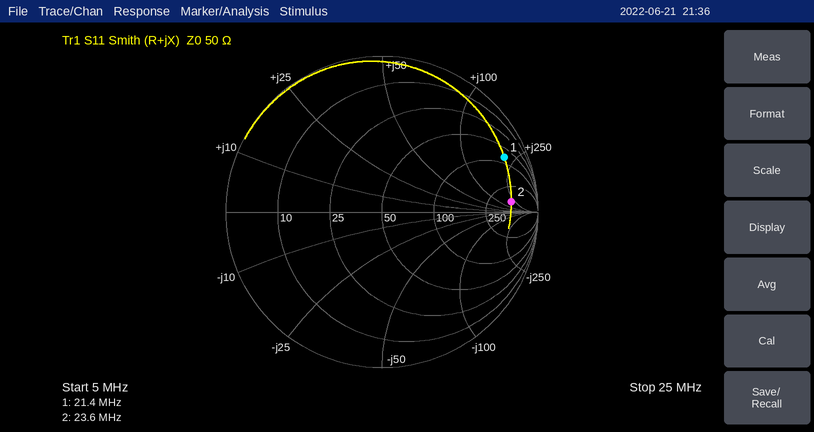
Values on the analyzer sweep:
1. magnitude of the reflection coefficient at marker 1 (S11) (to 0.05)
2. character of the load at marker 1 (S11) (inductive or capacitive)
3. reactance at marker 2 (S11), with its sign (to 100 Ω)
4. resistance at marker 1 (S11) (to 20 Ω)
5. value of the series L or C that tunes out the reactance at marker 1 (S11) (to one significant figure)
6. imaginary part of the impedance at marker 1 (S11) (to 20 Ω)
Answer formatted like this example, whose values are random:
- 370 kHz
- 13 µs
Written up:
- 0.85
- inductive
- +200 Ω
- 80 Ω
- 40 pF
- +200 Ω
